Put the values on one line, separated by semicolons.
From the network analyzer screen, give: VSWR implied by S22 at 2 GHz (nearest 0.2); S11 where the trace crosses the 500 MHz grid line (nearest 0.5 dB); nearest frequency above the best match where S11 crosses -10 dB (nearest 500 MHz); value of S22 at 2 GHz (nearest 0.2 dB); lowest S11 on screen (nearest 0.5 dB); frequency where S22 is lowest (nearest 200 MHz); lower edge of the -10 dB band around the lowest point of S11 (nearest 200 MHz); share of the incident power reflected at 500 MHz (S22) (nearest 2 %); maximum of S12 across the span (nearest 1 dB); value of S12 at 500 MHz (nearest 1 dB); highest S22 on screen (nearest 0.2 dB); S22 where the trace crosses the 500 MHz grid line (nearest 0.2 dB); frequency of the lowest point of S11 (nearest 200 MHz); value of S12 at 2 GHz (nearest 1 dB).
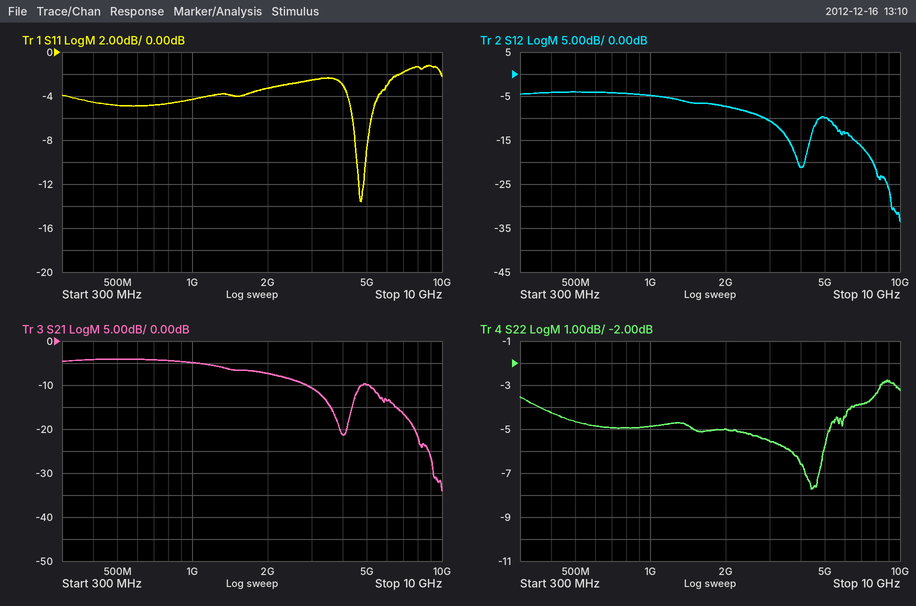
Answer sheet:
3.6; -5.0 dB; 5.0 GHz; -5.0 dB; -13.5 dB; 4.4 GHz; 4.6 GHz; 34 %; -4 dB; -4 dB; -2.8 dB; -4.6 dB; 4.8 GHz; -7 dB
